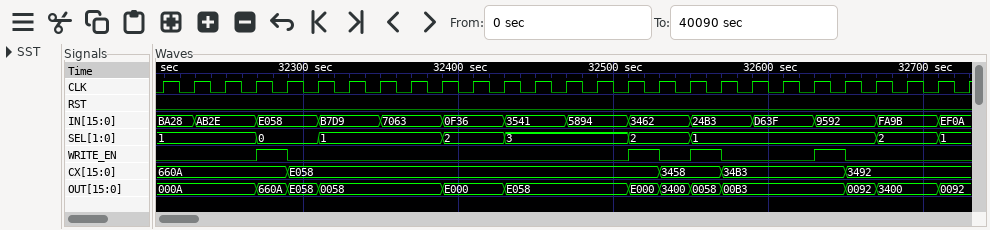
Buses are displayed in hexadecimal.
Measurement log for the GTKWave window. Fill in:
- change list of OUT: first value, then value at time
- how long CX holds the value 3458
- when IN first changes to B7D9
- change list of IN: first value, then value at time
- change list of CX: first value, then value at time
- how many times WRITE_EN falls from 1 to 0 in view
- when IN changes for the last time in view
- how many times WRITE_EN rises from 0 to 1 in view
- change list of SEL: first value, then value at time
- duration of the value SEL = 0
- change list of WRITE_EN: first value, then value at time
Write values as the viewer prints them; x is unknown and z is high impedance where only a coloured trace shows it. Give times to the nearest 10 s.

000A, 660A at 32270 s, E058 at 32290 s, 0058 at 32310 s, E000 at 32390 s, E058 at 32430 s, E000 at 32510 s, 3400 at 32530 s, 0058 at 32550 s, 00B3 at 32570 s, 0092 at 32650 s, 3400 at 32670 s, 0092 at 32710 s
40 s
32310 s
BA28, AB2E at 32230 s, E058 at 32270 s, B7D9 at 32310 s, 7063 at 32350 s, 0F36 at 32390 s, 3541 at 32430 s, 5894 at 32470 s, 3462 at 32510 s, 24B3 at 32550 s, D63F at 32590 s, 9592 at 32630 s, FA9B at 32670 s, EF0A at 32710 s
660A, E058 at 32290 s, 3458 at 32530 s, 34B3 at 32570 s, 3492 at 32650 s
4
32710 s
4
1, 0 at 32270 s, 1 at 32310 s, 2 at 32390 s, 3 at 32430 s, 2 at 32510 s, 1 at 32550 s, 2 at 32670 s, 1 at 32710 s
40 s
0, 1 at 32270 s, 0 at 32290 s, 1 at 32510 s, 0 at 32530 s, 1 at 32550 s, 0 at 32570 s, 1 at 32630 s, 0 at 32650 s
